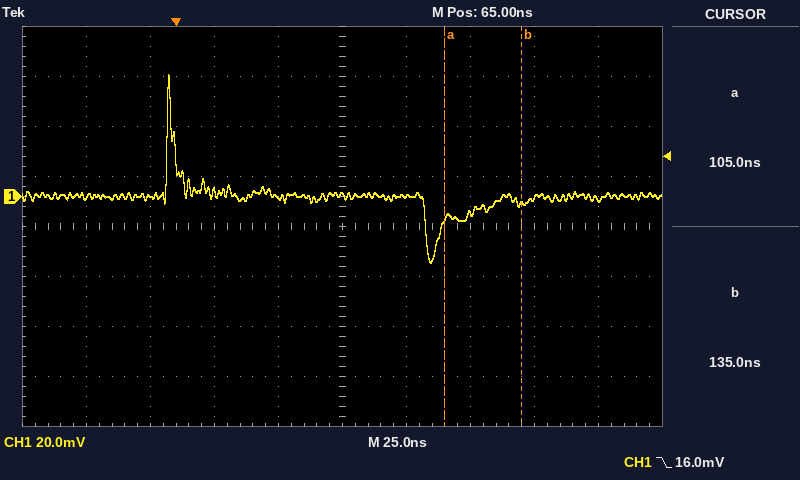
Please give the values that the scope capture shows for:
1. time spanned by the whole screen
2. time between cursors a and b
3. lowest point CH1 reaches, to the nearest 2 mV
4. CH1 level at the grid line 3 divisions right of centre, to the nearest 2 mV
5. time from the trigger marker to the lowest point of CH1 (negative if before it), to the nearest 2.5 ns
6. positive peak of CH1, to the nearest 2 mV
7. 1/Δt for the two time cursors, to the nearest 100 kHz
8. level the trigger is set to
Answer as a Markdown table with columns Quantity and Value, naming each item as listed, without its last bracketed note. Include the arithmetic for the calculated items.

| Quantity | Value |
|---|---|
| time spanned by the whole screen | 250 ns |
| time between cursors a and b | 135 ns − (105 ns) = 30.0 ns |
| lowest point CH1 reaches, to the nearest 2 mV | -26 mV |
| CH1 level at the grid line 3 divisions right of centre, to the nearest 2 mV | 0 mV |
| time from the trigger marker to the lowest point of CH1 (negative if before it), to the nearest 2.5 ns | +100.0 ns |
| positive peak of CH1, to the nearest 2 mV | 48 mV |
| 1/Δt for the two time cursors, to the nearest 100 kHz | 1 / 30.0 ns ≈ 33.3 MHz |
| level the trigger is set to | 16.0 mV |
